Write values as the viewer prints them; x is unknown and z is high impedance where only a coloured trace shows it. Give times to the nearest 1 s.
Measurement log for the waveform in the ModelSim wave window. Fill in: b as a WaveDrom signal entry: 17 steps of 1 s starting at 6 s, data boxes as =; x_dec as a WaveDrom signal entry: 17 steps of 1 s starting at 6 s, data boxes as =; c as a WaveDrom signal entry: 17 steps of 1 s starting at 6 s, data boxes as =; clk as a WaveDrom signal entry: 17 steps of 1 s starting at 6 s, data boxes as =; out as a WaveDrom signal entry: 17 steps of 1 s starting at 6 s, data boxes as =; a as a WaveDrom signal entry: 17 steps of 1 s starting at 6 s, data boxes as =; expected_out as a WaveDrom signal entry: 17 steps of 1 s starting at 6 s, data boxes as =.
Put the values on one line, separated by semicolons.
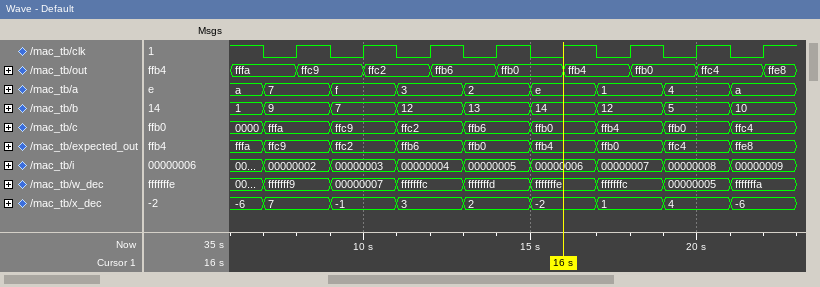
{name: 'b', wave: '==.=.=.=.=.=.=.=.', data: '1 9 7 12 13 14 12 5 10'}; {name: 'x_dec', wave: '==.=.=.=.=.=.=.=.', data: '-6 7 -1 3 2 -2 1 4 -6'}; {name: 'c', wave: '==.=.=.=.=.=.=.=.', data: '0000 fffa ffc9 ffc2 ffb6 ffb0 ffb4 ffb0 ffc4'}; {name: 'clk', wave: '10101010101010101'}; {name: 'out', wave: '=.=.=.=.=.=.=.=.=', data: 'fffa ffc9 ffc2 ffb6 ffb0 ffb4 ffb0 ffc4 ffe8'}; {name: 'a', wave: '==.=.=.=.=.=.=.=.', data: 'a 7 f 3 2 e 1 4 a'}; {name: 'expected_out', wave: '==.=.=.=.=.=.=.=.', data: 'fffa ffc9 ffc2 ffb6 ffb0 ffb4 ffb0 ffc4 ffe8'}
